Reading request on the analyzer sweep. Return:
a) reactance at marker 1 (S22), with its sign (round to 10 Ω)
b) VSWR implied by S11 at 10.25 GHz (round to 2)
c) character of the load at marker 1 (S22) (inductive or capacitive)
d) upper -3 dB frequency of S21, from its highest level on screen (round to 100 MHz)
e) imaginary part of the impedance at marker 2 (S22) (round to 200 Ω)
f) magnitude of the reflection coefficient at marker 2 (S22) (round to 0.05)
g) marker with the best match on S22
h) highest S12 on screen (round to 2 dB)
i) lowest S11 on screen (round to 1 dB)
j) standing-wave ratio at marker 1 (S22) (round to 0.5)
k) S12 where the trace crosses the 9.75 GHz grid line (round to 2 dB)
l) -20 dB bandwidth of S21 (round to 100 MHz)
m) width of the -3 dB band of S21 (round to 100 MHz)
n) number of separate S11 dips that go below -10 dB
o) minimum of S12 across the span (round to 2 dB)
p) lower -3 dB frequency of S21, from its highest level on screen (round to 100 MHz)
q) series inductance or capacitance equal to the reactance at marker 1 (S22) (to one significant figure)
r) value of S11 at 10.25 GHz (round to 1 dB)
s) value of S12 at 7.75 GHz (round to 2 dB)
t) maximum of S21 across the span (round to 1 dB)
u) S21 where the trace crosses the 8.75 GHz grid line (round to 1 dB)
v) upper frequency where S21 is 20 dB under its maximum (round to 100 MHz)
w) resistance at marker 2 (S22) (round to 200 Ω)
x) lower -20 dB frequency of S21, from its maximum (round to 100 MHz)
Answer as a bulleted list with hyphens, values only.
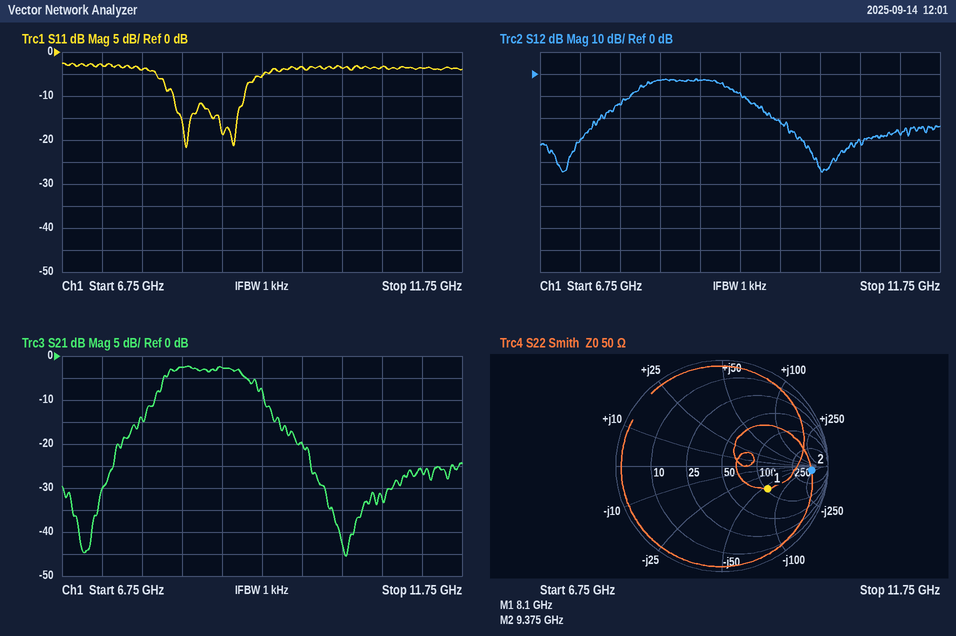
- -60 Ω
- 4
- capacitive
- 9.1 GHz
- -200 Ω
- 0.85
- marker 1
- -2 dB
- -22 dB
- 3.0
- -22 dB
- 2.4 GHz
- 1.1 GHz
- 2
- -44 dB
- 8.0 GHz
- 300 fF
- -4 dB
- -14 dB
- -2 dB
- -3 dB
- 9.8 GHz
- 600 Ω
- 7.4 GHz
